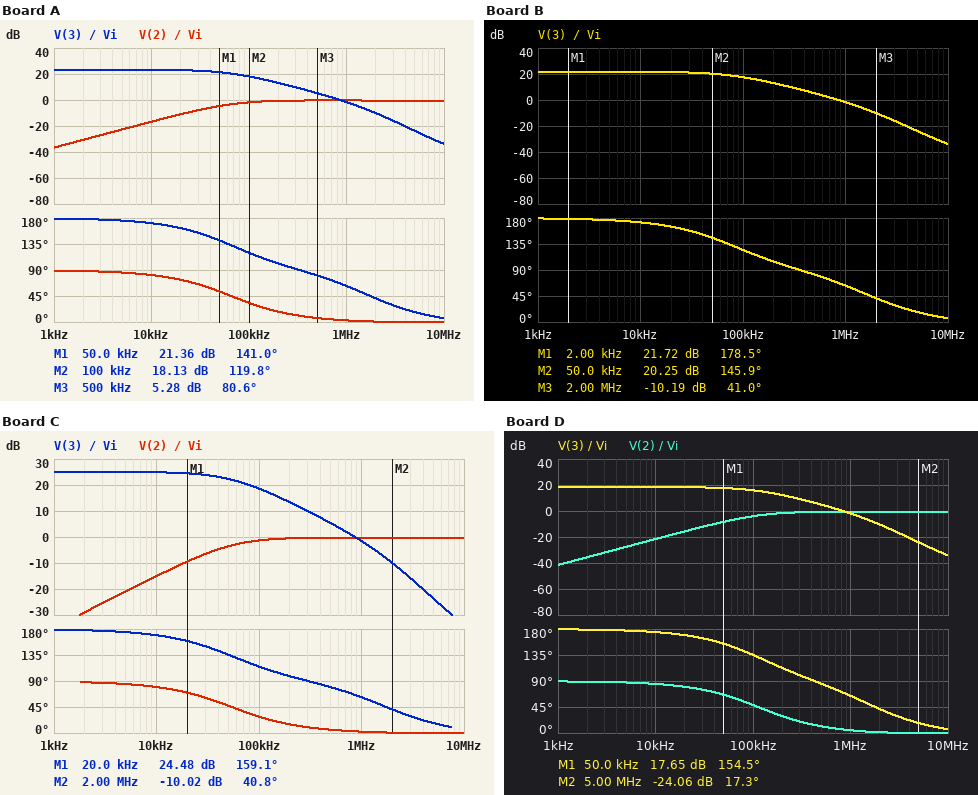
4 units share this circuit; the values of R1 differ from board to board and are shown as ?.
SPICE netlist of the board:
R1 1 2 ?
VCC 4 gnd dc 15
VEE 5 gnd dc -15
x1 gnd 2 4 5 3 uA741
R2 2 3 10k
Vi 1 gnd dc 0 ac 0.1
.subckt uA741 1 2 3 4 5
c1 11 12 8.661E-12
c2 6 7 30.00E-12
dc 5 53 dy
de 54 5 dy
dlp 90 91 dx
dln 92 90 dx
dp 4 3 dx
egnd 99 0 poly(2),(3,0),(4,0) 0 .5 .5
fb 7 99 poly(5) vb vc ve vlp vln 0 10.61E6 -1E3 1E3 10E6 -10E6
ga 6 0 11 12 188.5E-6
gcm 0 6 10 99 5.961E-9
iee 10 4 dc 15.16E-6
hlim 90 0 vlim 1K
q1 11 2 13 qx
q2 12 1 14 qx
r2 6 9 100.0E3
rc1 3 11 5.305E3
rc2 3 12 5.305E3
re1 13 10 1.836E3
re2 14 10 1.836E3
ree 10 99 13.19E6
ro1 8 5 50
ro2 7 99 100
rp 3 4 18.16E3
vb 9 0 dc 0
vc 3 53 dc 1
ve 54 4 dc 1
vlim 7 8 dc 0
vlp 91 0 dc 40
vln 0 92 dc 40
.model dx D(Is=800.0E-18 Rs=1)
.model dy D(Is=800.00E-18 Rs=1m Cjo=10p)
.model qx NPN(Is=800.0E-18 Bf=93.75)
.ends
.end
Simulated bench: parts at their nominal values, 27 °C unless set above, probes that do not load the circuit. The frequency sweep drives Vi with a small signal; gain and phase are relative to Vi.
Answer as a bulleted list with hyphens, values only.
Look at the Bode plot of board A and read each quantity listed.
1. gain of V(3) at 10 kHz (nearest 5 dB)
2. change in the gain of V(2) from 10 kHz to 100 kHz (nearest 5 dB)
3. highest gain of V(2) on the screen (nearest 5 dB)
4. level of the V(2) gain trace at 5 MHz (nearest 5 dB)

- 25 dB
- 15 dB
- 0 dB
- 0 dB
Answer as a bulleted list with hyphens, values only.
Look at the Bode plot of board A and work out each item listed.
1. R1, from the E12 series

- 680 Ω
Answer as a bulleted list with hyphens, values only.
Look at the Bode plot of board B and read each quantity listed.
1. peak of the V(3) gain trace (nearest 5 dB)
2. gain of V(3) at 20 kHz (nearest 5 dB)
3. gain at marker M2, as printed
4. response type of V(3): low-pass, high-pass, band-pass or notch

- 20 dB
- 20 dB
- 20.25 dB
- low-pass
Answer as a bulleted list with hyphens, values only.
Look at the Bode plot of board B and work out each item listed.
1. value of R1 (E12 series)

- 820 Ω
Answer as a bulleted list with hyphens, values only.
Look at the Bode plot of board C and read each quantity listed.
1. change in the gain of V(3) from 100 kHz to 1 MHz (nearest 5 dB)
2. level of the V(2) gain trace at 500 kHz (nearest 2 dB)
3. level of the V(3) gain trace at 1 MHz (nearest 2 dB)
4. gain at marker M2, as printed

- -20 dB
- 0 dB
- -2 dB
- -10.02 dB
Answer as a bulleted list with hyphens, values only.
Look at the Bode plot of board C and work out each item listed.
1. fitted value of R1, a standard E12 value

- 560 Ω
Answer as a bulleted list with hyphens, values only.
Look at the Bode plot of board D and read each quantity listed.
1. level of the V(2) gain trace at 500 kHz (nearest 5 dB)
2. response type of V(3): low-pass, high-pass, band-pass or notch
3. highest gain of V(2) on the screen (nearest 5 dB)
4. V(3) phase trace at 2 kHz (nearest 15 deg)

- 0 dB
- low-pass
- 0 dB
- 180 deg
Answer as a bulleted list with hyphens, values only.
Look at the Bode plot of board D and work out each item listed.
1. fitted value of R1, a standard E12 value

- 1.2 kΩ
